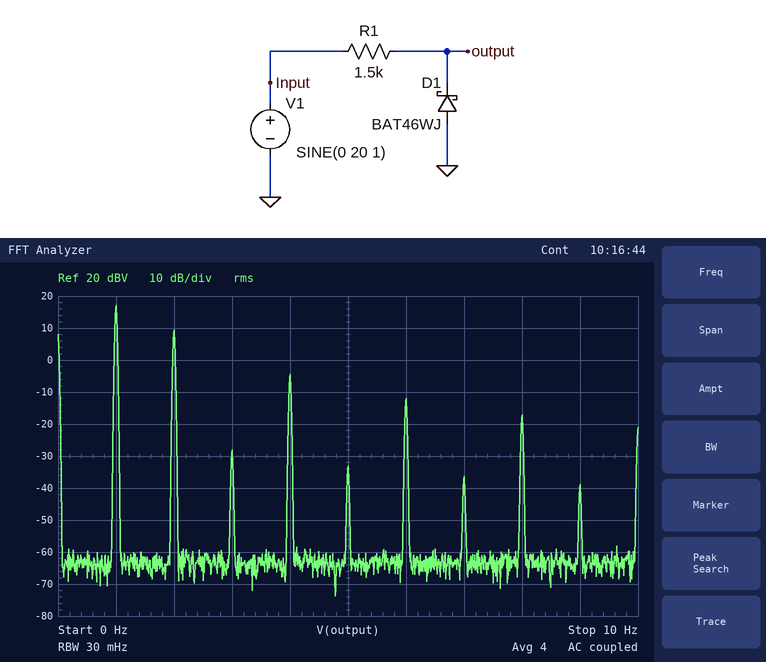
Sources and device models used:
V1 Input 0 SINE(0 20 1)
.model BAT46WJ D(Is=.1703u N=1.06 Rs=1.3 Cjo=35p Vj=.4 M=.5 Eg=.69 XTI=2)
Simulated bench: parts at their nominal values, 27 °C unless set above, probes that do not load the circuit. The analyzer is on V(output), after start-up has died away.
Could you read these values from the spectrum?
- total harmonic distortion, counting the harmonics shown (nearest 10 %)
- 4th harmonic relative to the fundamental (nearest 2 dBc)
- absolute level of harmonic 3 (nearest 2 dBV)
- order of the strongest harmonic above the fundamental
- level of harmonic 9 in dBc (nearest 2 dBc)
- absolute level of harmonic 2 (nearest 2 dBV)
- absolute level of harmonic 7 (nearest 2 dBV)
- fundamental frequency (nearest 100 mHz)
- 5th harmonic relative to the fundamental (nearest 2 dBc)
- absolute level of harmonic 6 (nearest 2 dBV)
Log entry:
40 %
-22 dBc
-28 dBV
2
-56 dBc
10 dBV
-36 dBV
1.0 Hz
-50 dBc
-12 dBV
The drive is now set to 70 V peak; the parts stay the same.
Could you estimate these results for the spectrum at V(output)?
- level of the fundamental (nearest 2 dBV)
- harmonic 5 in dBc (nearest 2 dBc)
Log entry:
28 dBV
-60 dBc
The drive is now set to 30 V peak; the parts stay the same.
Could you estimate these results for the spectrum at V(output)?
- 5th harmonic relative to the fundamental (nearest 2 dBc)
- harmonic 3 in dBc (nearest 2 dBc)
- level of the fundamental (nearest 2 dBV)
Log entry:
-54 dBc
-48 dBc
20 dBV
